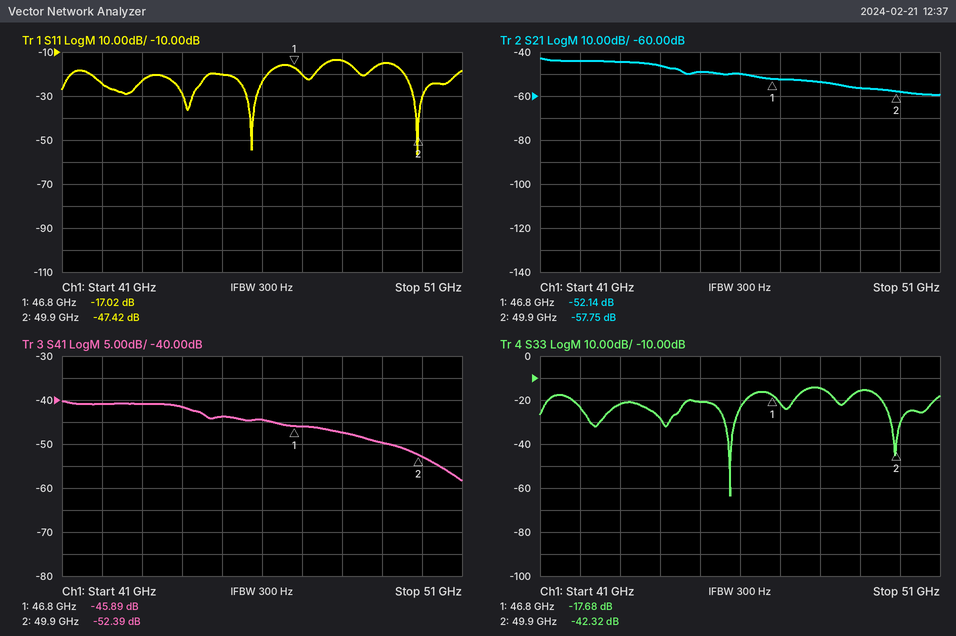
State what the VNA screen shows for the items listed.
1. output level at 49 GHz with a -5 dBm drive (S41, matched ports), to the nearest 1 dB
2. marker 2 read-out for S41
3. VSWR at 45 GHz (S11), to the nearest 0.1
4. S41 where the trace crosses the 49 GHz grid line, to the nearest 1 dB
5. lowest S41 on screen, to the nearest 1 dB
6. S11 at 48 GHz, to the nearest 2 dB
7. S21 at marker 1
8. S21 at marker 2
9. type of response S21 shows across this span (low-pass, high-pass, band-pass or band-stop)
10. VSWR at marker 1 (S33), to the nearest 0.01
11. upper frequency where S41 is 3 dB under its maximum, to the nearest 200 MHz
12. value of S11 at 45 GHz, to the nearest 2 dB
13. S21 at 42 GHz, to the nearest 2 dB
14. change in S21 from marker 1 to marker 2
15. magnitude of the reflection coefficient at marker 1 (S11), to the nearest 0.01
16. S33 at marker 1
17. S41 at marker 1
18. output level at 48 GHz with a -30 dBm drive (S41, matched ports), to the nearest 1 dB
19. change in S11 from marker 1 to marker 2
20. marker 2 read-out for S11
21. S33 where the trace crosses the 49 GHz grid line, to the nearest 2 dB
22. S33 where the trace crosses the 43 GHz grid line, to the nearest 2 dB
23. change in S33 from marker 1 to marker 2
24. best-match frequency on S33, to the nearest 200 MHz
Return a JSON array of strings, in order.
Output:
["-55 dBm", "-52.39 dB", "1.2", "-50 dB", "-58 dB", "-14 dB", "-52.14 dB", "-57.75 dB", "low-pass", "1.30", "44.6 GHz", "-20 dB", "-44 dB", "-5.61 dB", "0.14", "-17.68 dB", "-45.89 dB", "-77 dBm", "-30.40 dB", "-47.42 dB", "-16 dB", "-22 dB", "-24.64 dB", "45.8 GHz"]
